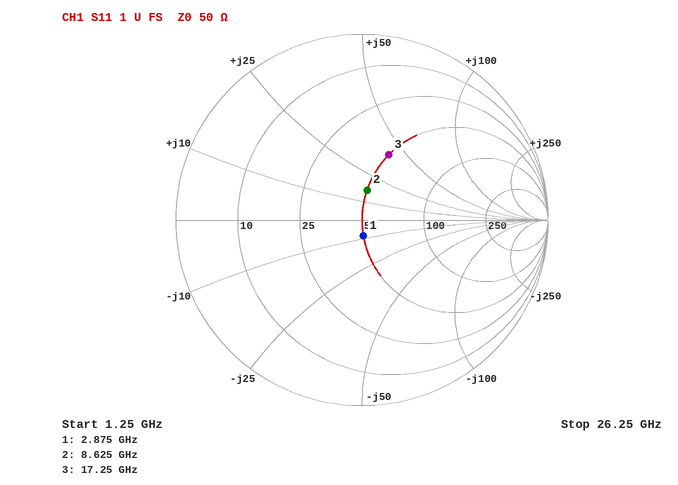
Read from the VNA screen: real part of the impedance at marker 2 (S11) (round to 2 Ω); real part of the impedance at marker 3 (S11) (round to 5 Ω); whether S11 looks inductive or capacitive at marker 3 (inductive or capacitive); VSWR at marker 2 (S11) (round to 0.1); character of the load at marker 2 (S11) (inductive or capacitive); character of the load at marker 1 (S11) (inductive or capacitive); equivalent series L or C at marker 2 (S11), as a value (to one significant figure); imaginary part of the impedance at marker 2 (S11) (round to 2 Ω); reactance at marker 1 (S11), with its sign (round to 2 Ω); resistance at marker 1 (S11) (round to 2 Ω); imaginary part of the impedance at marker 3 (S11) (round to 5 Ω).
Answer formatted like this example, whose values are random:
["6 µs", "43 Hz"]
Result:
["50 Ω", "50 Ω", "inductive", "1.4", "inductive", "capacitive", "300 pH", "+16 Ω", "-8 Ω", "50 Ω", "+40 Ω"]
